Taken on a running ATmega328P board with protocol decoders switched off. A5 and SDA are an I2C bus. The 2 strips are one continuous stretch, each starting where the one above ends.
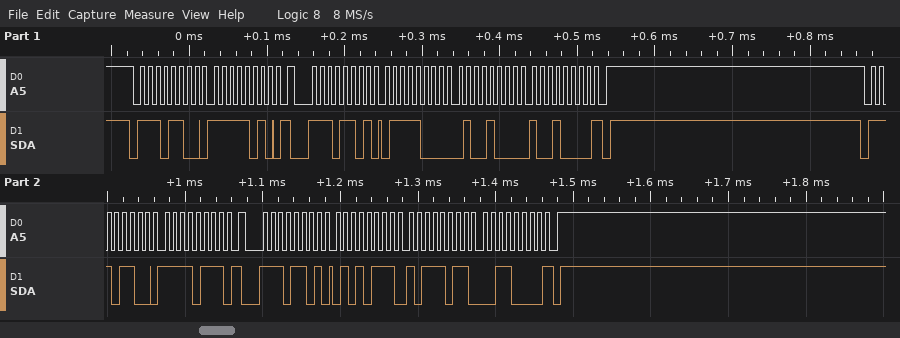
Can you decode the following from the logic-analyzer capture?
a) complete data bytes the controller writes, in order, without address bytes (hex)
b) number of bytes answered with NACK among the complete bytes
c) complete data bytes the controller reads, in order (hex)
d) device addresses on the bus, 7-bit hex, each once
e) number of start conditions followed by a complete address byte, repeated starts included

FA F7
2
78 48 90 57 BB 30
0x76
4
